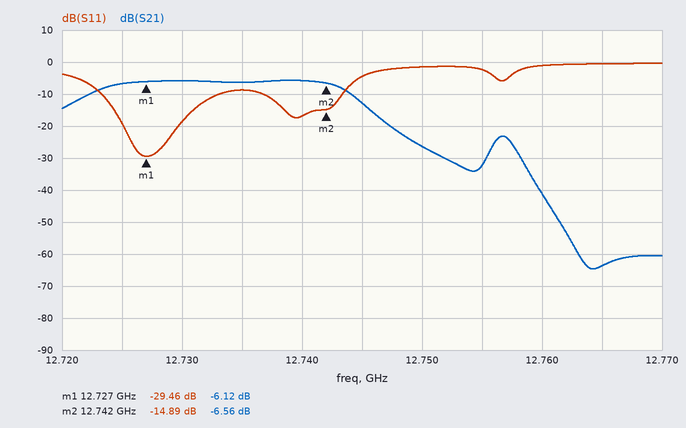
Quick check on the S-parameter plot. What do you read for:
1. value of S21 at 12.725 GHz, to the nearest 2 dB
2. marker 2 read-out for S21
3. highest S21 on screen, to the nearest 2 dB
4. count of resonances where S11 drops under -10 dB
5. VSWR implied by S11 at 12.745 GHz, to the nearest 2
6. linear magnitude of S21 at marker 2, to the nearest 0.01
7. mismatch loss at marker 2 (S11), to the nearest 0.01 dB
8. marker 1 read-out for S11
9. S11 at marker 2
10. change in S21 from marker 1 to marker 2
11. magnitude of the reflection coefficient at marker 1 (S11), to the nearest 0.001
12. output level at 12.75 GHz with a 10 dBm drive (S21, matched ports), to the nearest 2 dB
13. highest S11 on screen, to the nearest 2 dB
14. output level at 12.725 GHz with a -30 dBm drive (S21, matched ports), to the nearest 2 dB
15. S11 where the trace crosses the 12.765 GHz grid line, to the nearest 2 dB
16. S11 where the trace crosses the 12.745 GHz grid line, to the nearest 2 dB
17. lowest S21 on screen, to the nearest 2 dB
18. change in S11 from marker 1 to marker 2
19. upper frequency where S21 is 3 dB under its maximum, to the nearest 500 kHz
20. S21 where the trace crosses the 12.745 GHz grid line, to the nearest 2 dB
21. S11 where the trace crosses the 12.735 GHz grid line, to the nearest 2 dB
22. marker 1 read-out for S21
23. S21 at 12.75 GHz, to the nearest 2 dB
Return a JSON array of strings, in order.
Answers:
["-6 dB", "-6.56 dB", "-6 dB", "2", "4", "0.47", "0.14 dB", "-29.46 dB", "-14.89 dB", "-0.44 dB", "0.034", "-16 dBm", "0 dB", "-36 dBm", "0 dB", "-4 dB", "-64 dB", "14.57 dB", "12.7435 GHz", "-12 dB", "-8 dB", "-6.12 dB", "-26 dB"]
